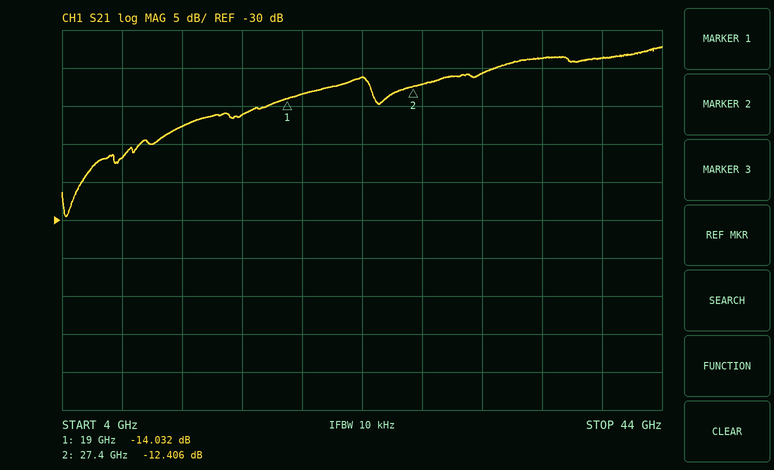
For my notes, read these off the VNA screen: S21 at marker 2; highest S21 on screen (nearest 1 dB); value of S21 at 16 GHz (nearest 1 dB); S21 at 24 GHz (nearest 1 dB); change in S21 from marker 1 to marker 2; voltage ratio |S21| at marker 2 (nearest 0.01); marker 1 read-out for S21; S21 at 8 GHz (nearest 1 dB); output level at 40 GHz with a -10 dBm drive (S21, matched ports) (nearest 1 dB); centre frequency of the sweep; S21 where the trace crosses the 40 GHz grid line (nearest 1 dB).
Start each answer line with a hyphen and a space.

- -12.406 dB
- -7 dB
- -16 dB
- -11 dB
- 1.626 dB
- 0.24
- -14.032 dB
- -22 dB
- -19 dBm
- 24 GHz
- -9 dB
